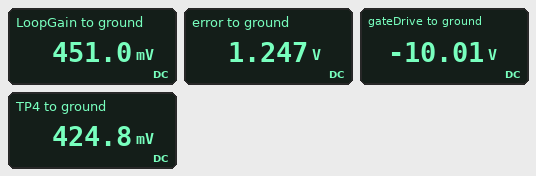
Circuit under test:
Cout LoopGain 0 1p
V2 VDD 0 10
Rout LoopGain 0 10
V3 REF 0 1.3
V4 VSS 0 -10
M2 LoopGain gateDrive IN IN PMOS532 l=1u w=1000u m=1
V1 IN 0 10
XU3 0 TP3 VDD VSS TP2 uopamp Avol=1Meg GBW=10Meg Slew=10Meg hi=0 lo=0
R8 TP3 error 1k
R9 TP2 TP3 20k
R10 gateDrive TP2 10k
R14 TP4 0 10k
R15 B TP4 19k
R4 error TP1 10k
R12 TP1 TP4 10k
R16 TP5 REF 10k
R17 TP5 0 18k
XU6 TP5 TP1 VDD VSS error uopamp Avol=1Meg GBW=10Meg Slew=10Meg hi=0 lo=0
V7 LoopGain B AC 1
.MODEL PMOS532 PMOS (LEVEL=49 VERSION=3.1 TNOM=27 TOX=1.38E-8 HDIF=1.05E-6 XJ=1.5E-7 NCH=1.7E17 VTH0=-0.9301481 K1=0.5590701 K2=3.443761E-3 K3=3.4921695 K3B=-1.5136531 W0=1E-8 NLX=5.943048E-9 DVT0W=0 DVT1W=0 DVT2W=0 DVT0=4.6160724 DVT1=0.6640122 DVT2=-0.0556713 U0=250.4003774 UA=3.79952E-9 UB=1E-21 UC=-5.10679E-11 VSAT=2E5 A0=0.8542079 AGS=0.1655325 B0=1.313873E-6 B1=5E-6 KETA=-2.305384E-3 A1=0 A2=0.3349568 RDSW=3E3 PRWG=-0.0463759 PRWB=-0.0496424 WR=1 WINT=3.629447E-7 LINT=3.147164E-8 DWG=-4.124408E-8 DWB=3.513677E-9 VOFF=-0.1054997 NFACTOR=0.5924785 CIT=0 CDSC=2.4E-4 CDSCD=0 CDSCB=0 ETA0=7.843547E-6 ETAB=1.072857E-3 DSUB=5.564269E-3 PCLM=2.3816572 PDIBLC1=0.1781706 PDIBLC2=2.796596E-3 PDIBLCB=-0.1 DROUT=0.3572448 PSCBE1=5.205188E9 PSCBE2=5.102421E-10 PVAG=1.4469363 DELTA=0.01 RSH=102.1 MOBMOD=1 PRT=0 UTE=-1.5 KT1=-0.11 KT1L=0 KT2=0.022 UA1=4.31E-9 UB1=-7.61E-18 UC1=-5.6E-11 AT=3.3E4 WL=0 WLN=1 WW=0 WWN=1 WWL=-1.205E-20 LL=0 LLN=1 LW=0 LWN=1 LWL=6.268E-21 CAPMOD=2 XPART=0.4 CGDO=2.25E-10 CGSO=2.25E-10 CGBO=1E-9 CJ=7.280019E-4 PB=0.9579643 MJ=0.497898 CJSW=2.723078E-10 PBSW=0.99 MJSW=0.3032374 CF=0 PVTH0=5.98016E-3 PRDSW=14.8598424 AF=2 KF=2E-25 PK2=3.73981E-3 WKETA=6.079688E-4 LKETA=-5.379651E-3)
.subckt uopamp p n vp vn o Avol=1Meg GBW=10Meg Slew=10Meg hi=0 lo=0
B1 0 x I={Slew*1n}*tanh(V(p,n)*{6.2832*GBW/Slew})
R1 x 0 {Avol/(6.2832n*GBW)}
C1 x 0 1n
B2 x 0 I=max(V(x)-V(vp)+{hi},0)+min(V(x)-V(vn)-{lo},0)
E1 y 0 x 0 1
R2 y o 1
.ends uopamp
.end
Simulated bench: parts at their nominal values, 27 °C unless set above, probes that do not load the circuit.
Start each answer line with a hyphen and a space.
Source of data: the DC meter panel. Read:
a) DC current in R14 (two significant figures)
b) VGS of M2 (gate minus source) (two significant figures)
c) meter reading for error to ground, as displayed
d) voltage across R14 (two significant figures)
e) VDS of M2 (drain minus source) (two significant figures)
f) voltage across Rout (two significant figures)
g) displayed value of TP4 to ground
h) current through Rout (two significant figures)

- 42 µA
- -20 V
- 1.247 V
- 420 mV
- -9.5 V
- 450 mV
- 424.8 mV
- 45 mA
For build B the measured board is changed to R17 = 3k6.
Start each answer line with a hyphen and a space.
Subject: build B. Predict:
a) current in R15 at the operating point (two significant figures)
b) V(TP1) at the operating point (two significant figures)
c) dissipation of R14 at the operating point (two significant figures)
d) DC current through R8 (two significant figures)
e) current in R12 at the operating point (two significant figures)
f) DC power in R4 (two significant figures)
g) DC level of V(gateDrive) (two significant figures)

- 12 µA
- 340 mV
- 5.3 µW
- 460 µA
- 11 µA
- 1.3 µW
- -9.2 V
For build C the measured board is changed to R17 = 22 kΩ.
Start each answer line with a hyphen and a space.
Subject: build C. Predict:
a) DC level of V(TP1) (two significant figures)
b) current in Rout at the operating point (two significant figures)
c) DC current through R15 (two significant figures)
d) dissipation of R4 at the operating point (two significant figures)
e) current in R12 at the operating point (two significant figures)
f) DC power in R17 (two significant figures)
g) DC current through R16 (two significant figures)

- 890 mV
- 45 mA
- 170 nA
- 20 µW
- 45 µA
- 36 µW
- 41 µA
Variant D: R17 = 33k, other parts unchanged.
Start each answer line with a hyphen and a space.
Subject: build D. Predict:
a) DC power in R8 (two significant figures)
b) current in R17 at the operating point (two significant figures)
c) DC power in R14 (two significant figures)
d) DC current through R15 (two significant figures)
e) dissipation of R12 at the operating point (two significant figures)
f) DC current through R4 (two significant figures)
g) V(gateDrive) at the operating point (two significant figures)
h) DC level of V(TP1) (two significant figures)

- 300 µW
- 30 µA
- 24 µW
- 2.0 µA
- 26 µW
- 51 µA
- -10 V
- 1.0 V
